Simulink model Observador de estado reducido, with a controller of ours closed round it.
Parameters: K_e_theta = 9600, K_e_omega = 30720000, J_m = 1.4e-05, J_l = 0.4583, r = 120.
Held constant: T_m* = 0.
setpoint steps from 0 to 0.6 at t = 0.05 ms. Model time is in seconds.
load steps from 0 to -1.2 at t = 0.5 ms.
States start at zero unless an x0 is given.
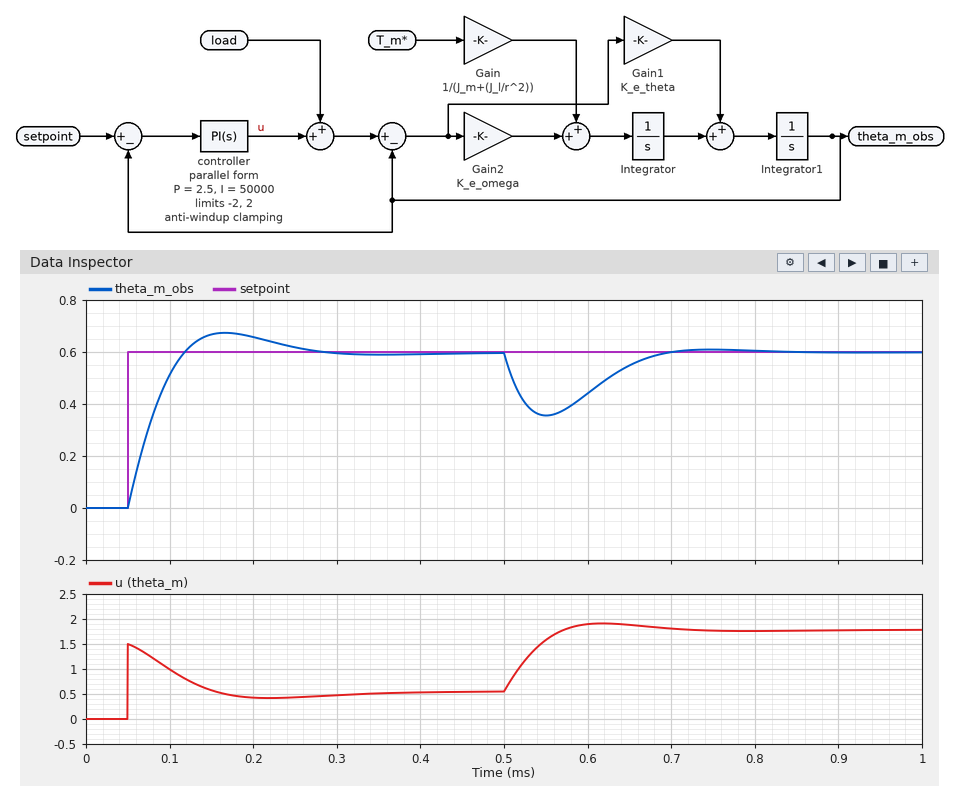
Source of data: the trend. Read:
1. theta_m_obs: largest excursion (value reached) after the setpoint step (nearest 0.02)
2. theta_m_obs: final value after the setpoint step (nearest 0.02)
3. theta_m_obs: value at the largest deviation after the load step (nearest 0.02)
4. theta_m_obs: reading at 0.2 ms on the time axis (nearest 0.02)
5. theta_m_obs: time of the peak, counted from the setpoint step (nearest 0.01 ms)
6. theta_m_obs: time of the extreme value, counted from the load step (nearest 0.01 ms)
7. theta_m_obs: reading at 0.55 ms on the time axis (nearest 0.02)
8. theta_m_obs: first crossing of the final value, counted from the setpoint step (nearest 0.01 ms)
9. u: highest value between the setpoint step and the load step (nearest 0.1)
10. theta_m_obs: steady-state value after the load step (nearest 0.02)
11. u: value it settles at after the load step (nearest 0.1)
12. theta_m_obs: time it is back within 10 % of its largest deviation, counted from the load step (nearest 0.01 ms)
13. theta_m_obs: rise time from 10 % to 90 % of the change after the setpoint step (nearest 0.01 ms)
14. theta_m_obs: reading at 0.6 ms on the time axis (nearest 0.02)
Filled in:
0.68
0.60
0.36
0.66
0.12 ms
0.05 ms
0.36
0.07 ms
1.5
0.60
1.8
0.17 ms
0.05 ms
0.44
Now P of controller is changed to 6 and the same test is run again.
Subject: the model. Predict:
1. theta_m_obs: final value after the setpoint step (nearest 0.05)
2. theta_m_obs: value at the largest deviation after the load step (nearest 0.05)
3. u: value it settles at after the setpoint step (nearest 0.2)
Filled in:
0.60
0.45
0.6
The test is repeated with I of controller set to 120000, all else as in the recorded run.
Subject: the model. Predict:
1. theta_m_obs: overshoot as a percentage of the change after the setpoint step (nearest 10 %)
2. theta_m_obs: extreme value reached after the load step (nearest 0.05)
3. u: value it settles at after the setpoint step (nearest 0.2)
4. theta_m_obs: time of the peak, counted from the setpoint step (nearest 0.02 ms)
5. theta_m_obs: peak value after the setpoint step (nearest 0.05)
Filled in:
30 %
0.40
0.6
0.08 ms
0.75
